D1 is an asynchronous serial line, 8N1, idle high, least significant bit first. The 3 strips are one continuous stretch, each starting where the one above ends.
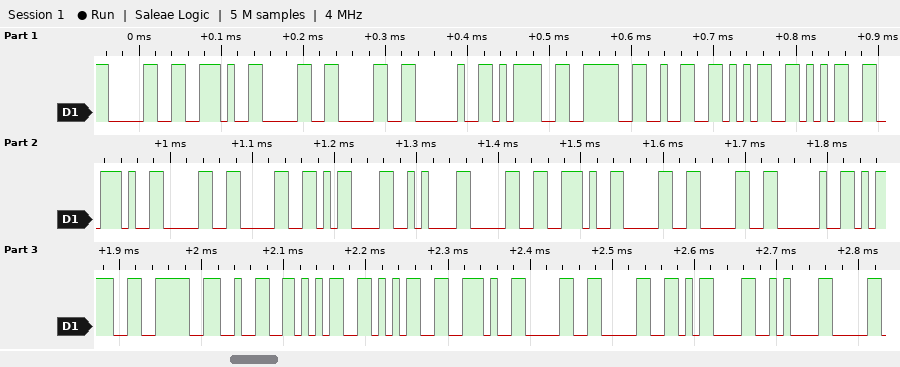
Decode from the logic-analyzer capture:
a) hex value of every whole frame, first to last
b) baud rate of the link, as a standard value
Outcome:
30 2E 30 30 20 3D 3E 32 35 35 2E 30 30 0D 0A 30 2E 30 30 20 3D 3E 32 35 35 2E 30 30 0D 0A
115200 baud
